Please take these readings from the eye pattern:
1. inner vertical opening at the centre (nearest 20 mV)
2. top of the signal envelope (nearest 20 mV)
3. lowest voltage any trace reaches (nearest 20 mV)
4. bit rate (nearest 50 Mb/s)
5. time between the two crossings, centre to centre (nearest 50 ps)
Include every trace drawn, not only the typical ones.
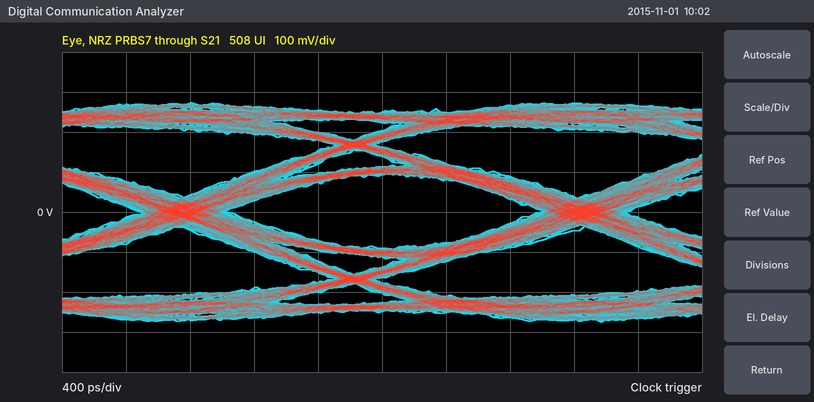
180 mV
280 mV
-280 mV
400 Mb/s
2.50 ns
